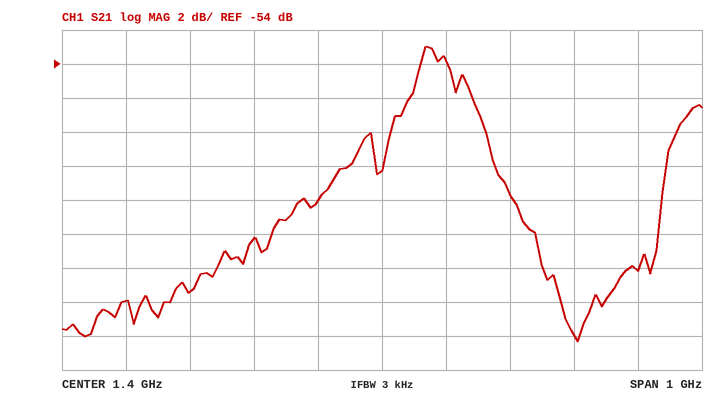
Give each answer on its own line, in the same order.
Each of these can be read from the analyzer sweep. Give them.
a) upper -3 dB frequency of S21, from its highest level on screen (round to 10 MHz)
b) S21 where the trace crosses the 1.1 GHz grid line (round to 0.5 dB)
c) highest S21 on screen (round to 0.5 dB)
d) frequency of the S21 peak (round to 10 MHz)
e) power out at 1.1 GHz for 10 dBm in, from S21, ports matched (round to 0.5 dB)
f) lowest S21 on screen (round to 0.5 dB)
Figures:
1.54 GHz
-67.5 dB
-53.0 dB
1.47 GHz
-57.5 dBm
-70.5 dB
